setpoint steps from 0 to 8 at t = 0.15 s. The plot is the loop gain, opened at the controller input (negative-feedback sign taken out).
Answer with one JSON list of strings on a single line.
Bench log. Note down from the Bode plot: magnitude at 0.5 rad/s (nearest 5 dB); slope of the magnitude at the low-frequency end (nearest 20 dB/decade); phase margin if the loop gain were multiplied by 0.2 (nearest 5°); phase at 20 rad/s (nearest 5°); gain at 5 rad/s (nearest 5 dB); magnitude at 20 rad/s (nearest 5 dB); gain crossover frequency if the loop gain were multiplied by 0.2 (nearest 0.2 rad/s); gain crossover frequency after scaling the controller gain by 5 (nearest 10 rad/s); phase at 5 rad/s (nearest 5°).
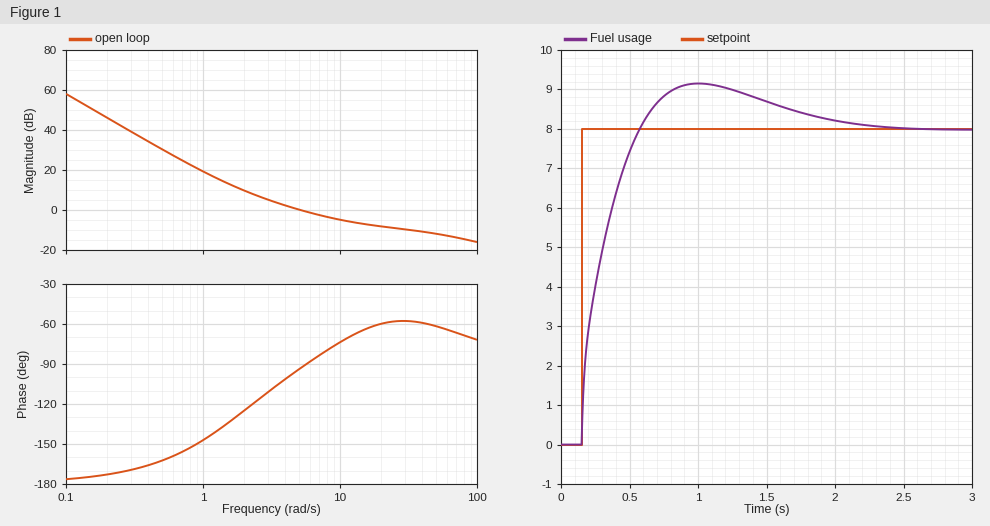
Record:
["30 dB", "-40 dB/decade", "45°", "-60°", "0 dB", "-10 dB", "1.4 rad/s", "70 rad/s", "-95°"]
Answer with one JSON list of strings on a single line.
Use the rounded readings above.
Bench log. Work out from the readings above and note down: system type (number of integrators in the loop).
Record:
["2"]
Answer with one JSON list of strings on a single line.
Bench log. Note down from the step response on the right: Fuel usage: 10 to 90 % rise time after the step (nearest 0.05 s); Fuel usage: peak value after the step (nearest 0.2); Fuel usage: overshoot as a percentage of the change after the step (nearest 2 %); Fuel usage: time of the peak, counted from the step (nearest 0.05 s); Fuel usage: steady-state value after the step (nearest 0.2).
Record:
["0.30 s", "9.2", "14 %", "0.85 s", "8.0"]
